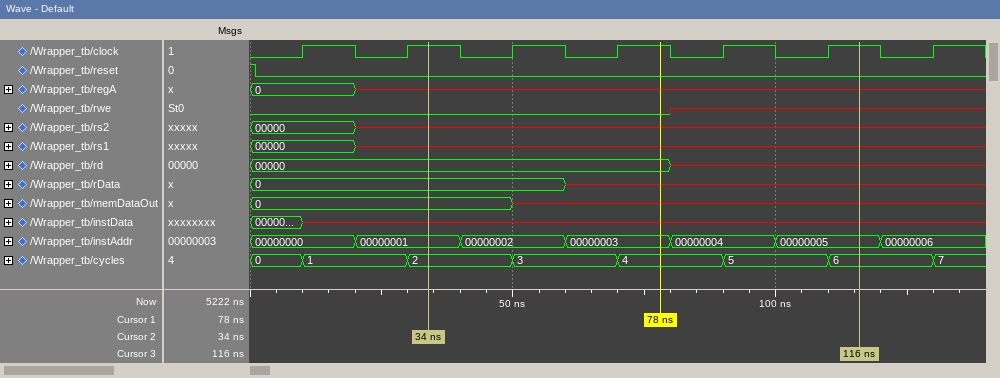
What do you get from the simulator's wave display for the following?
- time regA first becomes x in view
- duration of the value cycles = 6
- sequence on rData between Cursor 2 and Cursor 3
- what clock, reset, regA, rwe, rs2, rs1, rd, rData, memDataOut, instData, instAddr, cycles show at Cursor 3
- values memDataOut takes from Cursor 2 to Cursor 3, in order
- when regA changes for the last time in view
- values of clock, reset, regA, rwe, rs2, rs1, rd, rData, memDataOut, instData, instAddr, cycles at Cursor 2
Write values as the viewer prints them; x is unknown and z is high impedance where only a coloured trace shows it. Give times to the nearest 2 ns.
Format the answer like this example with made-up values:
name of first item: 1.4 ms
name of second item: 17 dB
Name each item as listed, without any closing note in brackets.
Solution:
time regA first becomes x in view: 20 ns
duration of the value cycles = 6: 20 ns
sequence on rData between Cursor 2 and Cursor 3: 0, x
what clock, reset, regA, rwe, rs2, rs1, rd, rData, memDataOut, instData, instAddr, cycles show at Cursor 3: clock=1, reset=0, regA=x, rwe=x, rs2=x, rs1=x, rd=x, rData=x, memDataOut=x, instData=x, instAddr=00000005, cycles=6
values memDataOut takes from Cursor 2 to Cursor 3, in order: 0, x
when regA changes for the last time in view: 20 ns
values of clock, reset, regA, rwe, rs2, rs1, rd, rData, memDataOut, instData, instAddr, cycles at Cursor 2: clock=1, reset=0, regA=x, rwe=0, rs2=x, rs1=x, rd=00000, rData=0, memDataOut=0, instData=x, instAddr=00000001, cycles=2
